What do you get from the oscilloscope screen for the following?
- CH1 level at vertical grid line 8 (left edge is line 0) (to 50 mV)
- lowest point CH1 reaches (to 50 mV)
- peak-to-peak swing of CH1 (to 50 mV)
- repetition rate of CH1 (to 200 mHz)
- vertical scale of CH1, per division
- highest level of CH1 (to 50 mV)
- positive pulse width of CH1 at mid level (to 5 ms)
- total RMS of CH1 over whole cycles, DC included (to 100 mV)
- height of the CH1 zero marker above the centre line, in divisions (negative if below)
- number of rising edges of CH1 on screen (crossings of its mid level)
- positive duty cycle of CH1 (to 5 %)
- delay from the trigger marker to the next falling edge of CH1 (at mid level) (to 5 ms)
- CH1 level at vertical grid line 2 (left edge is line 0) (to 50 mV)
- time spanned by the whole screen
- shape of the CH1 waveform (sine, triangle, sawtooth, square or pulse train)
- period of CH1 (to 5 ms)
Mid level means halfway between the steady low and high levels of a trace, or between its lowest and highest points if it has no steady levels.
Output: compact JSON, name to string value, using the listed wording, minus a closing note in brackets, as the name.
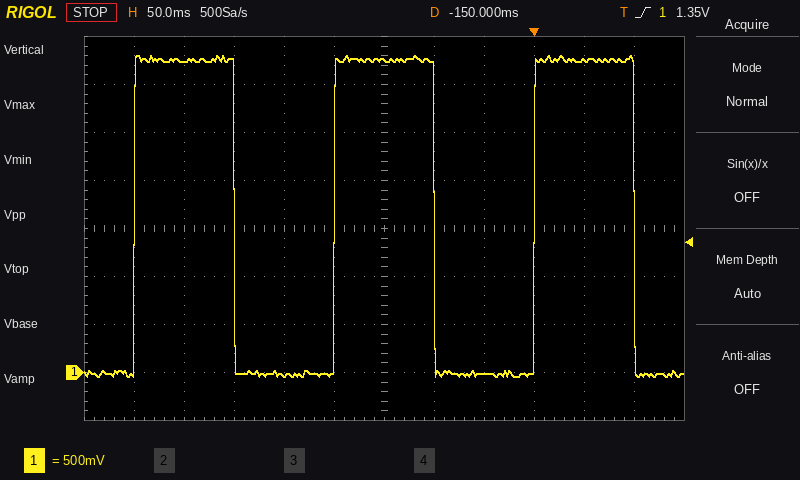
{"CH1 level at vertical grid line 8 (left edge is line 0)": "0 mV", "lowest point CH1 reaches": "-50 mV", "peak-to-peak swing of CH1": "3.35 V", "repetition rate of CH1": "5.0 Hz", "vertical scale of CH1, per division": "500 mV", "highest level of CH1": "3.30 V", "positive pulse width of CH1 at mid level": "100 ms", "total RMS of CH1 over whole cycles, DC included": "2.3 V", "height of the CH1 zero marker above the centre line, in divisions": "-3.0 div", "number of rising edges of CH1 on screen": "3", "positive duty cycle of CH1": "50 %", "delay from the trigger marker to the next falling edge of CH1 (at mid level)": "100 ms", "CH1 level at vertical grid line 2 (left edge is line 0)": "3.25 V", "time spanned by the whole screen": "600 ms", "shape of the CH1 waveform": "square", "period of CH1": "200 ms"}
